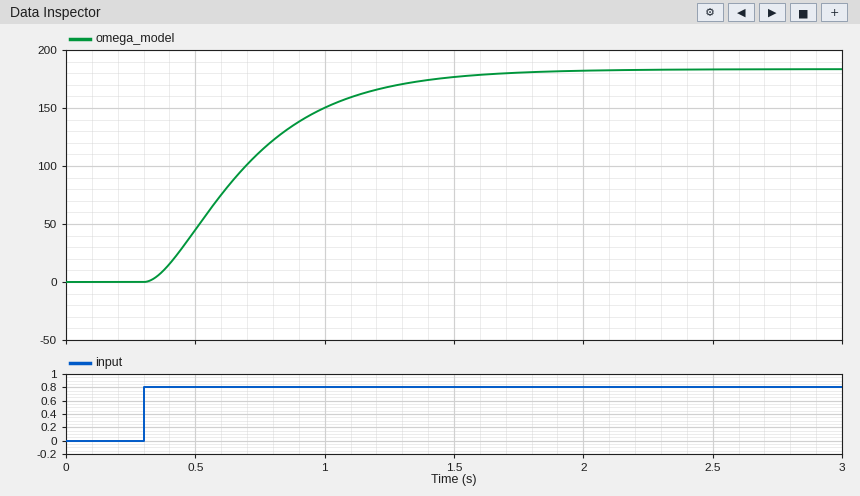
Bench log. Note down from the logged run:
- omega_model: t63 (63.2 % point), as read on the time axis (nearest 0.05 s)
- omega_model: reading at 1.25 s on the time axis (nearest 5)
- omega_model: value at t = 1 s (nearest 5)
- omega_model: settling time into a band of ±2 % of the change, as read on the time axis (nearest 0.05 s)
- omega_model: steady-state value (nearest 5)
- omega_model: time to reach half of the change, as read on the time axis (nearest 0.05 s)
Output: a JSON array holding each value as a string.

["0.75 s", "170", "150", "1.70 s", "185", "0.65 s"]
